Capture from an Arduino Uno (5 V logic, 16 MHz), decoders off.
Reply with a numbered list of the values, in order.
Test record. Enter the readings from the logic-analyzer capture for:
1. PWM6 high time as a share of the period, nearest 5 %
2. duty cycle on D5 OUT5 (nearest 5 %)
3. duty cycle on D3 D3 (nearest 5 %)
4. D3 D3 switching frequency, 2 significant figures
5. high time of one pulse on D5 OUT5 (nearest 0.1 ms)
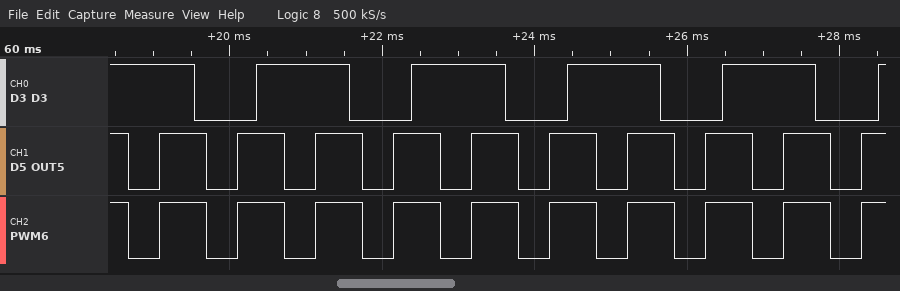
1. 60 %
2. 60 %
3. 60 %
4. 490 Hz
5. 0.6 ms
